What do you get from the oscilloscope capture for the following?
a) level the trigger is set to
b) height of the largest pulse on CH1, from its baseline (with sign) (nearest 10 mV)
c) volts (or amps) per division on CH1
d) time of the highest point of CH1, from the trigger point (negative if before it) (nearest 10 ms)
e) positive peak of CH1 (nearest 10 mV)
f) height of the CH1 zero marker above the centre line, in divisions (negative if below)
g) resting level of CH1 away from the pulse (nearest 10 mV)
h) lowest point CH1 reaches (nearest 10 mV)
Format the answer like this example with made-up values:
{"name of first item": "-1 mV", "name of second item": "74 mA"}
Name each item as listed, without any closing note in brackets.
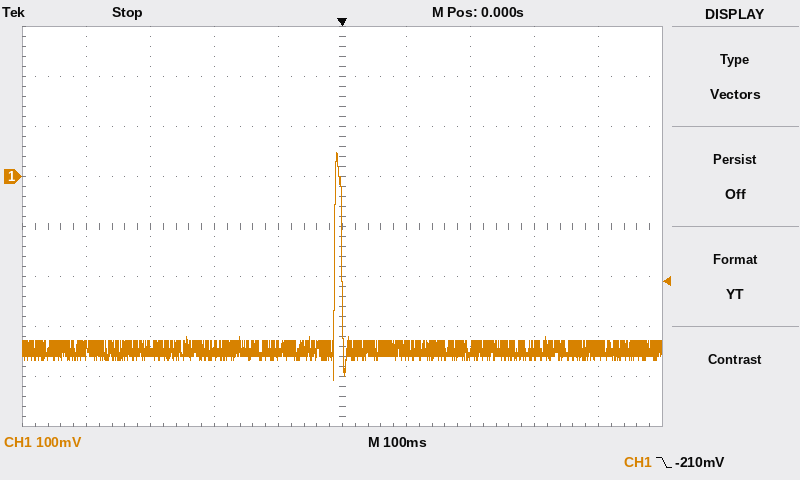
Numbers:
{"level the trigger is set to": "-210 mV", "height of the largest pulse on CH1, from its baseline (with sign)": "+390 mV", "volts (or amps) per division on CH1": "100 mV", "time of the highest point of CH1, from the trigger point (negative if before it)": "-10 ms", "positive peak of CH1": "50 mV", "height of the CH1 zero marker above the centre line, in divisions": "+1.0 div", "resting level of CH1 away from the pulse": "-340 mV", "lowest point CH1 reaches": "-410 mV"}
